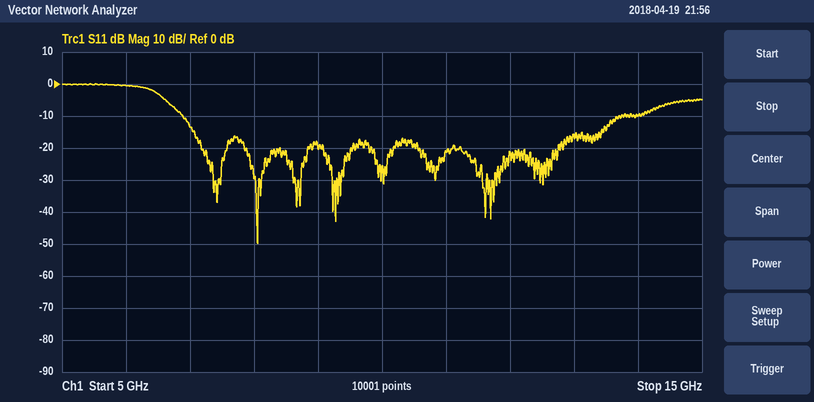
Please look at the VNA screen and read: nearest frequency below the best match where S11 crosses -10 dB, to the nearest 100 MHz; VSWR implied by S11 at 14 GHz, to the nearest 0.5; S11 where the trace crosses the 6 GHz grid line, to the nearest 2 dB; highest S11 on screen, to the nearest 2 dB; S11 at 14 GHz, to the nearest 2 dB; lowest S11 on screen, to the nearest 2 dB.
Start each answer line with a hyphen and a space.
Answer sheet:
- 6.9 GHz
- 2.0
- 0 dB
- 0 dB
- -10 dB
- -50 dB
